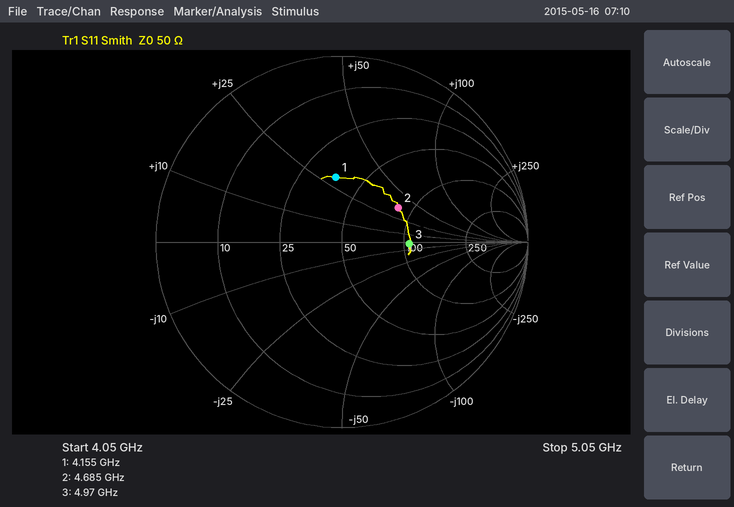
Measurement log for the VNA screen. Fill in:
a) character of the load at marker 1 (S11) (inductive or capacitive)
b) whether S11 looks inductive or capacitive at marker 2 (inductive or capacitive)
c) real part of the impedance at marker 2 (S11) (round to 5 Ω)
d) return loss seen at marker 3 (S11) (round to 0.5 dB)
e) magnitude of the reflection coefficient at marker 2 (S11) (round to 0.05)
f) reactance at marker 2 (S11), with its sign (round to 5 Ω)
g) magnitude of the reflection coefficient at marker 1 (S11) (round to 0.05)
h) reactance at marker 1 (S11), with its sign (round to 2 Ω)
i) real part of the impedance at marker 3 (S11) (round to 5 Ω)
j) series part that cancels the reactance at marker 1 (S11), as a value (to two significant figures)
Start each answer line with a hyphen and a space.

- inductive
- inductive
- 85 Ω
- 9.0 dB
- 0.35
- +35 Ω
- 0.35
- +30 Ω
- 105 Ω
- 1.3 pF
